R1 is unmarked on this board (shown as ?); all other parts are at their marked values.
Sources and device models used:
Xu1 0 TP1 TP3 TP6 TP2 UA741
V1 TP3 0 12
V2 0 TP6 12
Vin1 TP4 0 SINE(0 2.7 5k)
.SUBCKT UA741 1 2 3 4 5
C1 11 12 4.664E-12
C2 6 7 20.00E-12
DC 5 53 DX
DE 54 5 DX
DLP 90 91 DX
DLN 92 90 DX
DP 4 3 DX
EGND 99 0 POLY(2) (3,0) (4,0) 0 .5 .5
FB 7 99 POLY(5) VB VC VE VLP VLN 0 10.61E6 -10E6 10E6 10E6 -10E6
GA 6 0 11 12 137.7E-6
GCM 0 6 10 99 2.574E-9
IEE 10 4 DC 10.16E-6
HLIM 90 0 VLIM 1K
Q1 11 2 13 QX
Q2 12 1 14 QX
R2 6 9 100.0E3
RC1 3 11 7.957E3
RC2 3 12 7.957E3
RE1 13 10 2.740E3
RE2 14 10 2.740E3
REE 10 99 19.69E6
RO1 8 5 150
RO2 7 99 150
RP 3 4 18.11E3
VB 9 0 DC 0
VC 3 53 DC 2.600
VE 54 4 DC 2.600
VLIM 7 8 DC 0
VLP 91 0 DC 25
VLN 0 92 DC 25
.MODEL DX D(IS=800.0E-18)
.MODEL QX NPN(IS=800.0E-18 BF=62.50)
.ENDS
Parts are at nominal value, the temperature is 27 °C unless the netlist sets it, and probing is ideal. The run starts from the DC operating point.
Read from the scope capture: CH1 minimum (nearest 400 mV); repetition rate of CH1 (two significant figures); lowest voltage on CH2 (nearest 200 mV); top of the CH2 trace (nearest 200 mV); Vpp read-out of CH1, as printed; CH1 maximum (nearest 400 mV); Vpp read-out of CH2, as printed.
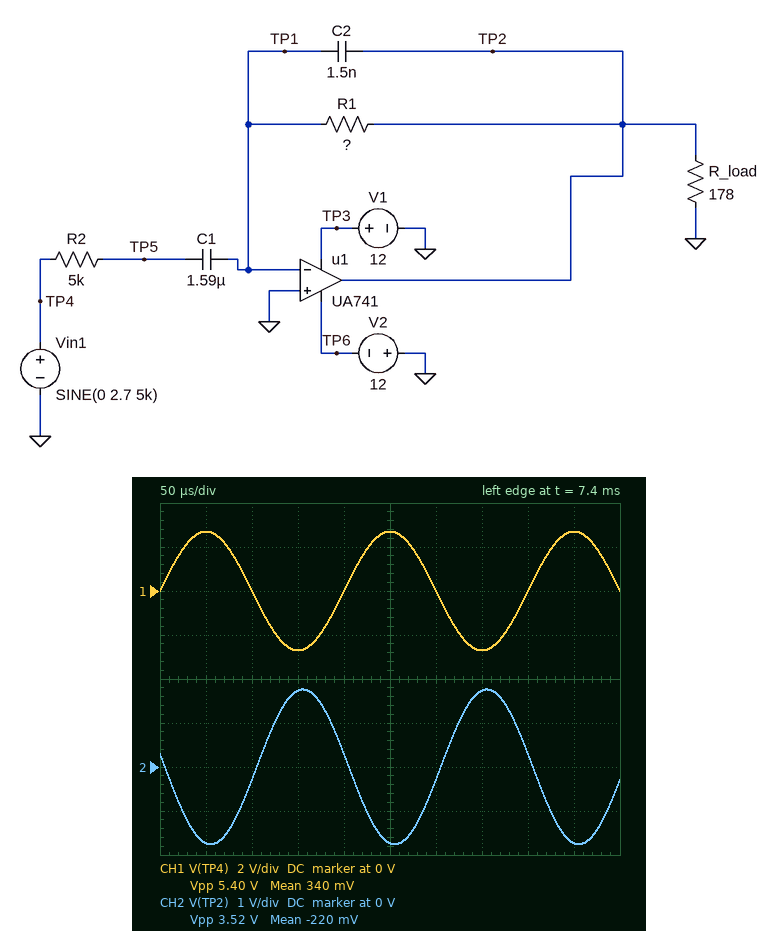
-2.8 V
5.0 kHz
-1.8 V
1.8 V
5.40 V
2.8 V
3.52 V
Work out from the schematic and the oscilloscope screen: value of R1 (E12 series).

3.3 kΩ
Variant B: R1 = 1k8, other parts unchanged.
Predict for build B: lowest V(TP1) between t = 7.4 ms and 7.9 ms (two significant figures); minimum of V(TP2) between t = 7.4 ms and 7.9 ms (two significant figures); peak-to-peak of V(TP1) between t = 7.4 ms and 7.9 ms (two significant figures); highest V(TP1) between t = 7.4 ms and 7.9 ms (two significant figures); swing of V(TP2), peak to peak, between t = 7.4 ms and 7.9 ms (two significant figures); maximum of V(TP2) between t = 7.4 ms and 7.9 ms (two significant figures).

-8.5 mV
-970 mV
17 mV
8.6 mV
1.9 V
970 mV
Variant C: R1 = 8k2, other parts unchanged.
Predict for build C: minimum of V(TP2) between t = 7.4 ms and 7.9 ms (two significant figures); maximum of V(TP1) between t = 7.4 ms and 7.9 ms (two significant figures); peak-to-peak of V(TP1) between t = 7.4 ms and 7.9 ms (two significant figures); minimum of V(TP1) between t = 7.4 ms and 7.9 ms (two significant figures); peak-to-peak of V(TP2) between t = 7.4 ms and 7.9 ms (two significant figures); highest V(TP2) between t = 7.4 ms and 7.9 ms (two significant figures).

-4.1 V
37 mV
73 mV
-37 mV
8.2 V
4.1 V
